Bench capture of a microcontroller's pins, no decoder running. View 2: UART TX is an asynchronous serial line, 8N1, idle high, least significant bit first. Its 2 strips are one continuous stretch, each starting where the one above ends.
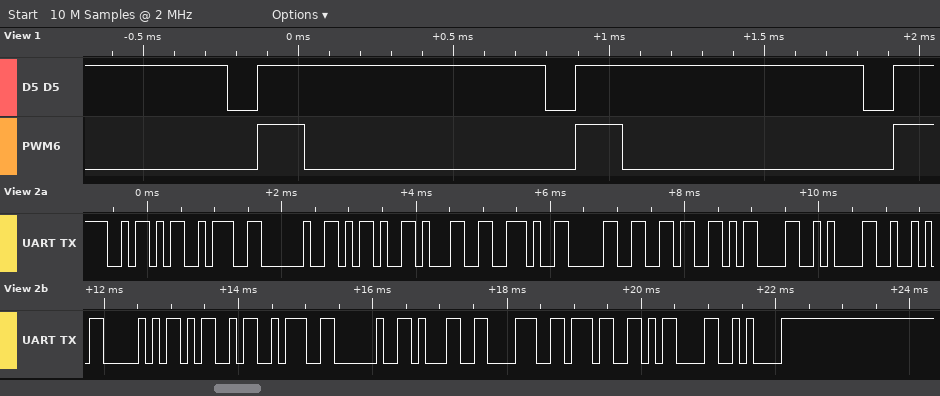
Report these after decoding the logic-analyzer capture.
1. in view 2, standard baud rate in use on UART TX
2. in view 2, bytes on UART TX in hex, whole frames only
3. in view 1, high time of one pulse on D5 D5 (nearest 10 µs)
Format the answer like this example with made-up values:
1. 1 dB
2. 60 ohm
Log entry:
1. 9600 baud
2. 5A 3A 20 2D 31 2E 30 36 0D 0A 52 50 4D 3A 20 31 38 37 0D 0A
3. 930 µs
